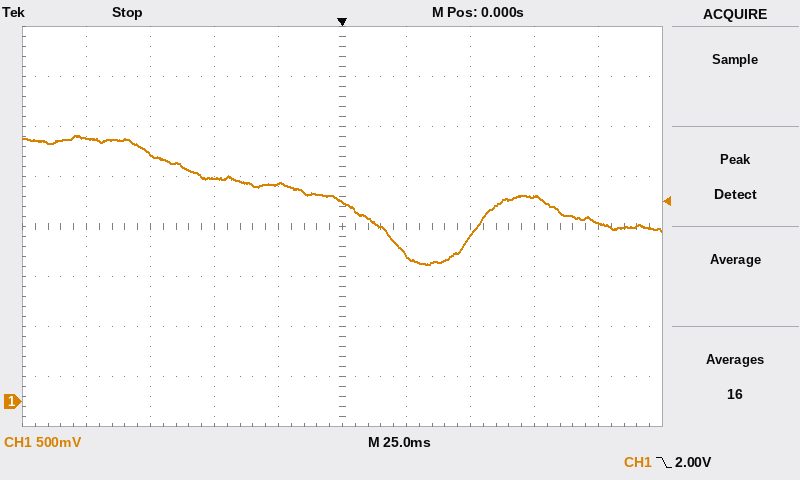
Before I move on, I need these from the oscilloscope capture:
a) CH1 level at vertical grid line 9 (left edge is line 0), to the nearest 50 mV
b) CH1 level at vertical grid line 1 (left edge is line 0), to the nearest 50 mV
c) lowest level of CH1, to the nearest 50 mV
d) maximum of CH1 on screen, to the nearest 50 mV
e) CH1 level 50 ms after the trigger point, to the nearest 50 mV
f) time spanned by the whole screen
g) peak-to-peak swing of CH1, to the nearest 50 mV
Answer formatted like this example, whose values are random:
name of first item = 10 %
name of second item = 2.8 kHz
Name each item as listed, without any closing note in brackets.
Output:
CH1 level at vertical grid line 9 (left edge is line 0), to the nearest 50 mV = 1.80 V
CH1 level at vertical grid line 1 (left edge is line 0), to the nearest 50 mV = 2.65 V
lowest level of CH1, to the nearest 50 mV = 1.35 V
maximum of CH1 on screen, to the nearest 50 mV = 2.65 V
CH1 level 50 ms after the trigger point, to the nearest 50 mV = 1.65 V
time spanned by the whole screen = 250 ms
peak-to-peak swing of CH1, to the nearest 50 mV = 1.30 V
